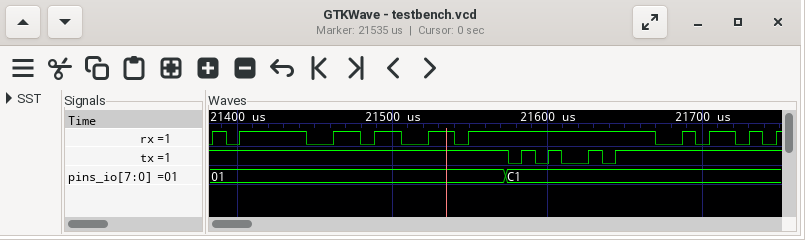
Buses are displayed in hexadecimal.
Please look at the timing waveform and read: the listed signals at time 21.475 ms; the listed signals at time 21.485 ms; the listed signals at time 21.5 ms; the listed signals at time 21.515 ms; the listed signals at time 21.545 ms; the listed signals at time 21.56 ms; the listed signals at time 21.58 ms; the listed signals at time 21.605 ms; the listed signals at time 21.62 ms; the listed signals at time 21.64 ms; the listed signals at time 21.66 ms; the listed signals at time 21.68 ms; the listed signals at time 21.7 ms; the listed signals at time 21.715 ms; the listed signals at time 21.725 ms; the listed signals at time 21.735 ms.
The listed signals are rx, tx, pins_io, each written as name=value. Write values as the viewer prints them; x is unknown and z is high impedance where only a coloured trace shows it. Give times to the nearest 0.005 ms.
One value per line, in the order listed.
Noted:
rx=1, tx=1, pins_io=01
rx=0, tx=1, pins_io=01
rx=1, tx=1, pins_io=01
rx=0, tx=1, pins_io=01
rx=0, tx=1, pins_io=01
rx=1, tx=1, pins_io=01
rx=1, tx=0, pins_io=C1
rx=1, tx=1, pins_io=C1
rx=1, tx=0, pins_io=C1
rx=1, tx=0, pins_io=C1
rx=1, tx=1, pins_io=C1
rx=0, tx=1, pins_io=C1
rx=0, tx=1, pins_io=C1
rx=1, tx=1, pins_io=C1
rx=0, tx=1, pins_io=C1
rx=1, tx=1, pins_io=C1
